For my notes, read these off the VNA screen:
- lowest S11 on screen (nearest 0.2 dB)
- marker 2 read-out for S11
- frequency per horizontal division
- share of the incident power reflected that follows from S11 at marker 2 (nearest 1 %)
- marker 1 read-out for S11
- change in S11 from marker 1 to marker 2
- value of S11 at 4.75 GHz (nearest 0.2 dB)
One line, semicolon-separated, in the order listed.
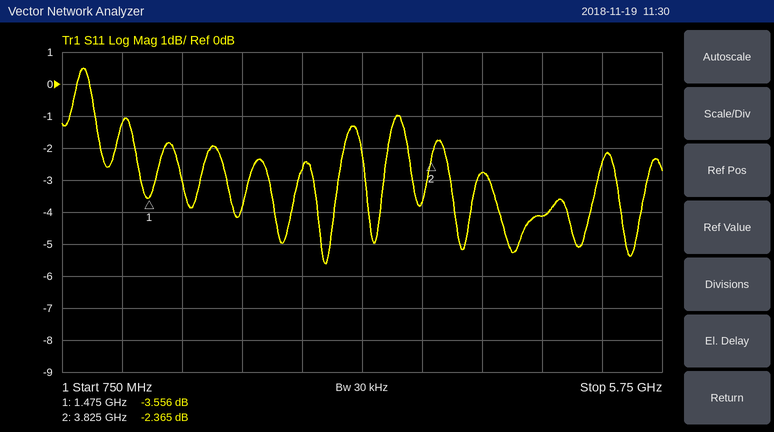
-5.6 dB; -2.365 dB; 500 MHz; 58 %; -3.556 dB; 1.191 dB; -4.2 dB
